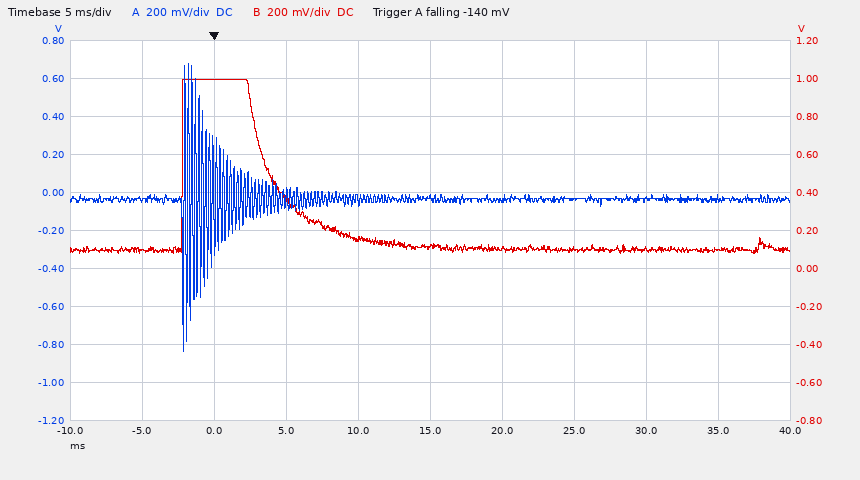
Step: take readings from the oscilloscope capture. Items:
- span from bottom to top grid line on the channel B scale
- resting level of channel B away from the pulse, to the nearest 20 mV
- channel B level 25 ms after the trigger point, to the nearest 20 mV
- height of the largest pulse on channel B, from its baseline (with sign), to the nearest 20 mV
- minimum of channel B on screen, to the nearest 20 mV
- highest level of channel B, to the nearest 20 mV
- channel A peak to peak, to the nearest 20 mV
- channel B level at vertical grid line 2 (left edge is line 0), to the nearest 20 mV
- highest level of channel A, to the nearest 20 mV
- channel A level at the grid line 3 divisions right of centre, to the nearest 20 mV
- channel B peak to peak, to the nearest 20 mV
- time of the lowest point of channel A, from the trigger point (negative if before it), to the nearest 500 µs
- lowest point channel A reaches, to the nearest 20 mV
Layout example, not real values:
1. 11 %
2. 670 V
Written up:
1. 2 V
2. 100 mV
3. 100 mV
4. +900 mV
5. 80 mV
6. 1.00 V
7. 1.52 V
8. 1.00 V
9. 680 mV
10. -40 mV
11. 920 mV
12. -2.0 ms
13. -840 mV
